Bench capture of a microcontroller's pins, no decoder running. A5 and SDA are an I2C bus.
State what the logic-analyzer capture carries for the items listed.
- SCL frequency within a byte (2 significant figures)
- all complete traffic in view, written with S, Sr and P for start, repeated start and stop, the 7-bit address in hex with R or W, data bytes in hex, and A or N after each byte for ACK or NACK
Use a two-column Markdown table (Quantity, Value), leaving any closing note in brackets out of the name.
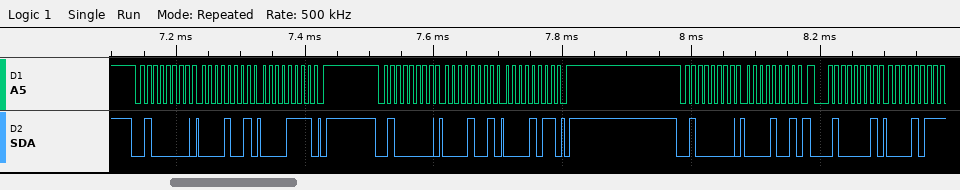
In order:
| Quantity | Value |
|---|---|
| SCL frequency within a byte | 100 kHz |
| all complete traffic in view, written with S, Sr and P for start, repeated start and stop, the 7-bit address in hex with R or W, data bytes in hex, and A or N after each byte for ACK or NACK | S 20W A 09 A 0F A P S 20W A 09 A 0B A P S 20W A 09 A Sr 20R A 0B N |
